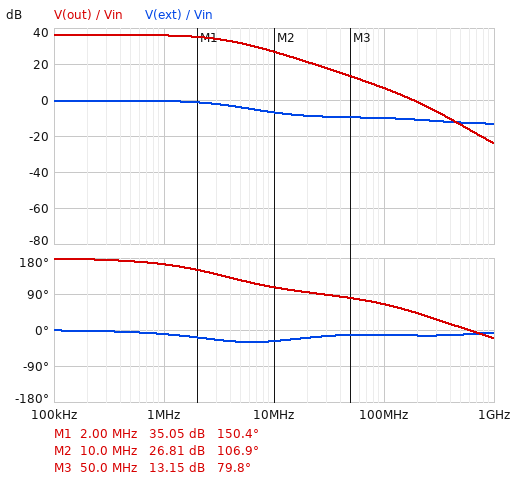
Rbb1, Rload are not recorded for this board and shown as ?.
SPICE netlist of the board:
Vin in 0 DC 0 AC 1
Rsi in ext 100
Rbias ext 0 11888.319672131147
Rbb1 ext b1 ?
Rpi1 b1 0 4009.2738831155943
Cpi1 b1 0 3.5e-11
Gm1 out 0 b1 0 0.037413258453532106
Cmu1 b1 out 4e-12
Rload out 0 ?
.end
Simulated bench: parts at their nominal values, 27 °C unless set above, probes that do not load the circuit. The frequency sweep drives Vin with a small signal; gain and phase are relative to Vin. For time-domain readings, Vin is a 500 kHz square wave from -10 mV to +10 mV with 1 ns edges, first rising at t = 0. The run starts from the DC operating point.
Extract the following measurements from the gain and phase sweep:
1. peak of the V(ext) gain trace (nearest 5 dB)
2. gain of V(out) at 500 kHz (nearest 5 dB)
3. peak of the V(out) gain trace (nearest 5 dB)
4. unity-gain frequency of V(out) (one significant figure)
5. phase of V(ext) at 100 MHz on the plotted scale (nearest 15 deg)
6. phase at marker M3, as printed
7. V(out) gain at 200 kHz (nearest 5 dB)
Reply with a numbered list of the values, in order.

1. 0 dB
2. 35 dB
3. 35 dB
4. 200 MHz
5. -15 deg
6. 79.8 deg
7. 35 dB
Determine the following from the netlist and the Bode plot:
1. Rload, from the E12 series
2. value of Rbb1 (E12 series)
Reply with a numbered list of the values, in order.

1. 1.8 kΩ
2. 27 Ω
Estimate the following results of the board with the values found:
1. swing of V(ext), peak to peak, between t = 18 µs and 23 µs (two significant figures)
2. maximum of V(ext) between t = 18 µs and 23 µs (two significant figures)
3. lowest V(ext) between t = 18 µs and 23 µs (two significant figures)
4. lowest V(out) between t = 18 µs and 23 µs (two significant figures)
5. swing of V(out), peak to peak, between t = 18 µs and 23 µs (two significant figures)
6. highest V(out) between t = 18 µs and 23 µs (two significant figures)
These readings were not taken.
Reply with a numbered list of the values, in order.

1. 19 mV
2. 9.7 mV
3. -9.7 mV
4. -650 mV
5. 1.3 V
6. 650 mV
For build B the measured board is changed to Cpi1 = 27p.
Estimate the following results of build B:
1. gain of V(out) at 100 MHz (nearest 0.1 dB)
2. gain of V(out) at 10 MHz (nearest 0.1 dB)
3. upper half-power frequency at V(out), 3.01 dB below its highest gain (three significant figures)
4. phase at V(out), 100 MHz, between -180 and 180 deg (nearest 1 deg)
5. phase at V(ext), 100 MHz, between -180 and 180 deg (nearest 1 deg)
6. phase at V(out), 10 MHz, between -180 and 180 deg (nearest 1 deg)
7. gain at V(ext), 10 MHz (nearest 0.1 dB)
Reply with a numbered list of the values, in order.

1. 7.0 dB
2. 27.0 dB
3. 3.67 MHz
4. 69 deg
5. -11 deg
6. 108 deg
7. -6.8 dB
